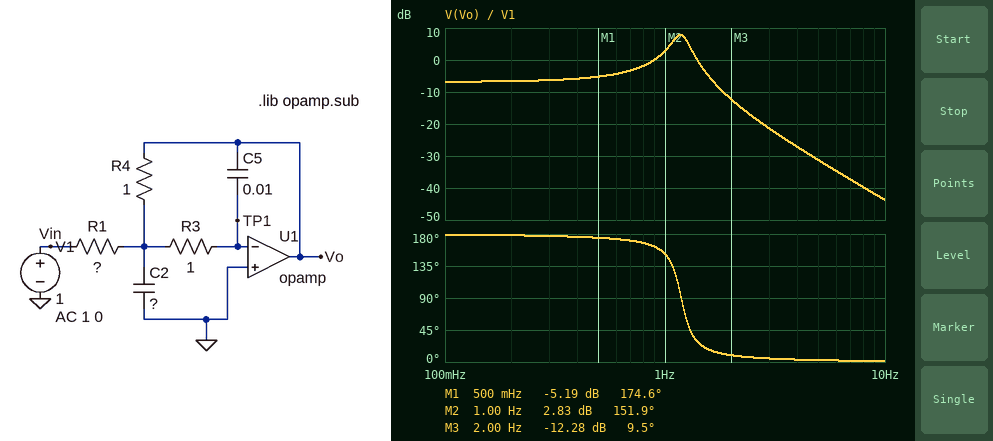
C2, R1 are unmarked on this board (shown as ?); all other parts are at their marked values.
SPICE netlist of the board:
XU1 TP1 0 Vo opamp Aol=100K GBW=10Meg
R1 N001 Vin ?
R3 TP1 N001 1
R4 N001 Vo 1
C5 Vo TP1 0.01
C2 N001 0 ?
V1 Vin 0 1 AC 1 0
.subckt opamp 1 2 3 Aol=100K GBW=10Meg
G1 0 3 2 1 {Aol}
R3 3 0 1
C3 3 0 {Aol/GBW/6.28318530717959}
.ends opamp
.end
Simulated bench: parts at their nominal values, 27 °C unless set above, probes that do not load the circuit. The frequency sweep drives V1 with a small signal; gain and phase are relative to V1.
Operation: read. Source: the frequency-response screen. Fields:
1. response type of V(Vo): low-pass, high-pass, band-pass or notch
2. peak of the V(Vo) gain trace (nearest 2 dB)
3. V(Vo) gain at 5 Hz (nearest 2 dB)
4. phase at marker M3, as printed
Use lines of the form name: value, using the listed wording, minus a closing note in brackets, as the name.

response type of V(Vo): low-pass, high-pass, band-pass or notch: low-pass
peak of the V(Vo) gain trace: 8 dB
V(Vo) gain at 5 Hz: -32 dB
phase at marker M3, as printed: 9.5 deg
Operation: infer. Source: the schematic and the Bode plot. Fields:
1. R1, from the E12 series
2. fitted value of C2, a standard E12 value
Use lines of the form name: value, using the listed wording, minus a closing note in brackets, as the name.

R1, from the E12 series: 2.2 Ω
fitted value of C2, a standard E12 value: 1.8 F
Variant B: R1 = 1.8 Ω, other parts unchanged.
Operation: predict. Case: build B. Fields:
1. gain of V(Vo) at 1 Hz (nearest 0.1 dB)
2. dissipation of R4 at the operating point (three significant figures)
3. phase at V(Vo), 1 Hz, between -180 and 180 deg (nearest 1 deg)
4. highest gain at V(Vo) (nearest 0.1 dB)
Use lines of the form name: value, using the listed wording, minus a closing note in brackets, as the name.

gain of V(Vo) at 1 Hz: 4.5 dB
dissipation of R4 at the operating point: 309 mW
phase at V(Vo), 1 Hz, between -180 and 180 deg: 151 deg
highest gain at V(Vo): 9.3 dB
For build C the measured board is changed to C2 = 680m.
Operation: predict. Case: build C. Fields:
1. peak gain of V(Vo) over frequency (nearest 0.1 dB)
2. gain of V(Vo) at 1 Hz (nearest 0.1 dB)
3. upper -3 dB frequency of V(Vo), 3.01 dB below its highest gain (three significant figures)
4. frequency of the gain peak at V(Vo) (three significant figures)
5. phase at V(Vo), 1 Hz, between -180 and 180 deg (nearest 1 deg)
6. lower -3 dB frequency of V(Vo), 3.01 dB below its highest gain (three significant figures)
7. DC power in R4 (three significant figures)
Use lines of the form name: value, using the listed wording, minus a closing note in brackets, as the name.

peak gain of V(Vo) over frequency: 3.8 dB
gain of V(Vo) at 1 Hz: -4.3 dB
upper -3 dB frequency of V(Vo), 3.01 dB below its highest gain: 2.16 Hz
frequency of the gain peak at V(Vo): 1.89 Hz
phase at V(Vo), 1 Hz, between -180 and 180 deg: 168 deg
lower -3 dB frequency of V(Vo), 3.01 dB below its highest gain: 1.57 Hz
DC power in R4: 207 mW
